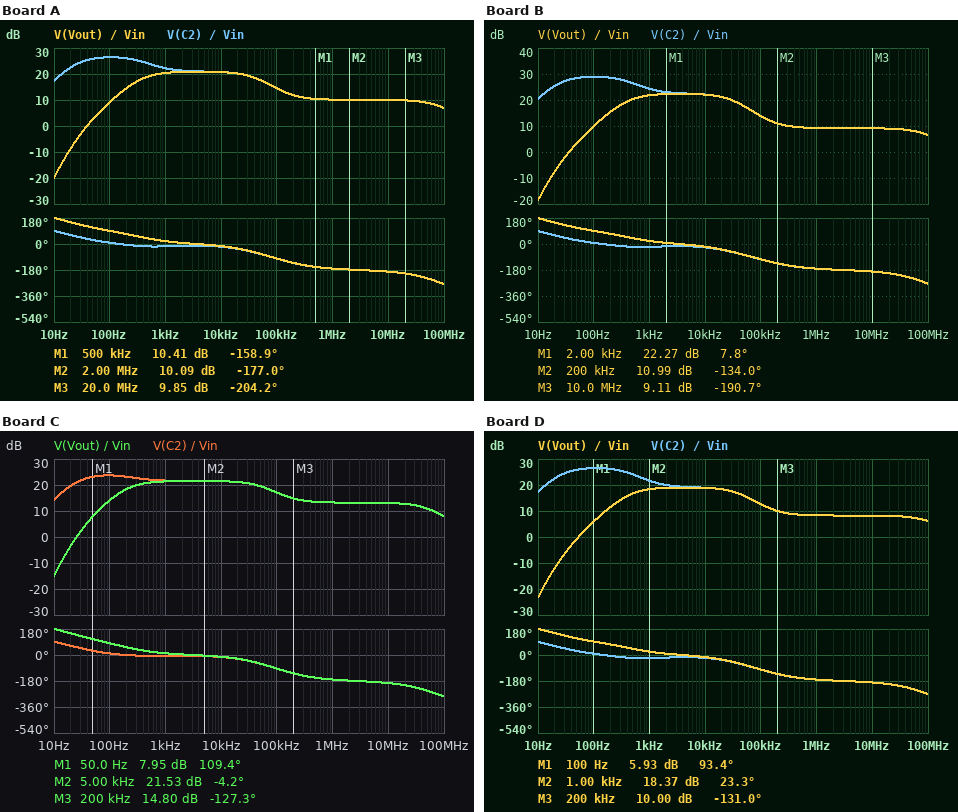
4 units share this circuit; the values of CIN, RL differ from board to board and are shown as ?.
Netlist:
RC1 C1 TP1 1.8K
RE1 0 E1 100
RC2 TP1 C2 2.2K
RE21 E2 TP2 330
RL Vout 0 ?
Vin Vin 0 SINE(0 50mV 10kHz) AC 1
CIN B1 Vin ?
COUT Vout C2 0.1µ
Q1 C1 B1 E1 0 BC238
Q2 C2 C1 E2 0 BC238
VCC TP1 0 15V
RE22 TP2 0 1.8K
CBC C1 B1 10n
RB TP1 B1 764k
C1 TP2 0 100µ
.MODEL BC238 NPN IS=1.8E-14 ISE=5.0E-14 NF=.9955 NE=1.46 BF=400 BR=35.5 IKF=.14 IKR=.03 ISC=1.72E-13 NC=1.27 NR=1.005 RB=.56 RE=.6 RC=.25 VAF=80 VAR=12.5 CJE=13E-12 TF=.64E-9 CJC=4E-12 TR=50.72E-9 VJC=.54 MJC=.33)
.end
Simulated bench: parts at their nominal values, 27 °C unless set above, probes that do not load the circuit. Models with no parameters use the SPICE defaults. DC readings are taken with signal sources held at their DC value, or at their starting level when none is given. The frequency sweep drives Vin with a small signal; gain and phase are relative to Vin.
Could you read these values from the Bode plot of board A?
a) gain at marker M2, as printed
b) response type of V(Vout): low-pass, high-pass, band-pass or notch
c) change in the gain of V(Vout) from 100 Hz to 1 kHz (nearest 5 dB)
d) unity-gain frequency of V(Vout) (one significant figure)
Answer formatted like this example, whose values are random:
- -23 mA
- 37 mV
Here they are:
- 10.09 dB
- band-pass
- 10 dB
- 40 Hz
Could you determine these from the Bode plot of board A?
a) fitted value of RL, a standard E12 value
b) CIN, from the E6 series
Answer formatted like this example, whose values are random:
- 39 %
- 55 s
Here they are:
- 2.2 kΩ
- 47 nF
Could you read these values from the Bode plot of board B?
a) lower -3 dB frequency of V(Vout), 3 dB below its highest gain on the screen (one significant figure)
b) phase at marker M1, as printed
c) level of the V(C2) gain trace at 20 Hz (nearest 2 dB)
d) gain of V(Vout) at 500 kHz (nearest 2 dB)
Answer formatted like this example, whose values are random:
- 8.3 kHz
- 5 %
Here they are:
- 400 Hz
- 7.8 deg
- 26 dB
- 10 dB
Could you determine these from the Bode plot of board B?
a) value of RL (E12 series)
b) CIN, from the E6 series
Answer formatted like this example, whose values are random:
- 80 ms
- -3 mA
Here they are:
- 1.8 kΩ
- 68 nF
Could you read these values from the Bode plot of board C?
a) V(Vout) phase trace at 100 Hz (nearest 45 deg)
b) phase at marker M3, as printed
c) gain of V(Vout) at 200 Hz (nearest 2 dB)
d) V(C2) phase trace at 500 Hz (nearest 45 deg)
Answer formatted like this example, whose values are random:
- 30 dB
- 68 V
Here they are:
- 90 deg
- -127.3 deg
- 18 dB
- 0 deg
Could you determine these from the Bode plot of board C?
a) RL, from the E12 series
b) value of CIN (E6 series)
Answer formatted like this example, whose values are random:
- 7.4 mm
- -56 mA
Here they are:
- 5.6 kΩ
- 33 nF
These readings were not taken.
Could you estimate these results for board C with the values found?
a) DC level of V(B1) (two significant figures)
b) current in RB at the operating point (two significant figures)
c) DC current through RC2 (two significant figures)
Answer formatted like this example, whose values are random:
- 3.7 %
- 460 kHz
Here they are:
- 1.2 V
- 18 µA
- 2.0 mA
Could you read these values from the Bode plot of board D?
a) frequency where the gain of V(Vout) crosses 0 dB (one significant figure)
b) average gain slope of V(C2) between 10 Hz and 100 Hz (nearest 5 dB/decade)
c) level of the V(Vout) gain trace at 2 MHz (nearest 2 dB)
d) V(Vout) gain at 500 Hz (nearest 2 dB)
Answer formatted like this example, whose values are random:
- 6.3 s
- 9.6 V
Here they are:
- 50 Hz
- 10 dB/decade
- 8 dB
- 16 dB
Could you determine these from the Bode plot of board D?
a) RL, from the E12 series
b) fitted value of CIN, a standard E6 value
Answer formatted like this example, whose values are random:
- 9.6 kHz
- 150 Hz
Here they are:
- 1.5 kΩ
- 47 nF
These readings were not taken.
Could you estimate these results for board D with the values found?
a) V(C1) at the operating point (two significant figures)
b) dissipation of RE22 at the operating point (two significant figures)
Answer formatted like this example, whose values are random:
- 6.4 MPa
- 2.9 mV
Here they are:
- 5.0 V
- 7.6 mW
